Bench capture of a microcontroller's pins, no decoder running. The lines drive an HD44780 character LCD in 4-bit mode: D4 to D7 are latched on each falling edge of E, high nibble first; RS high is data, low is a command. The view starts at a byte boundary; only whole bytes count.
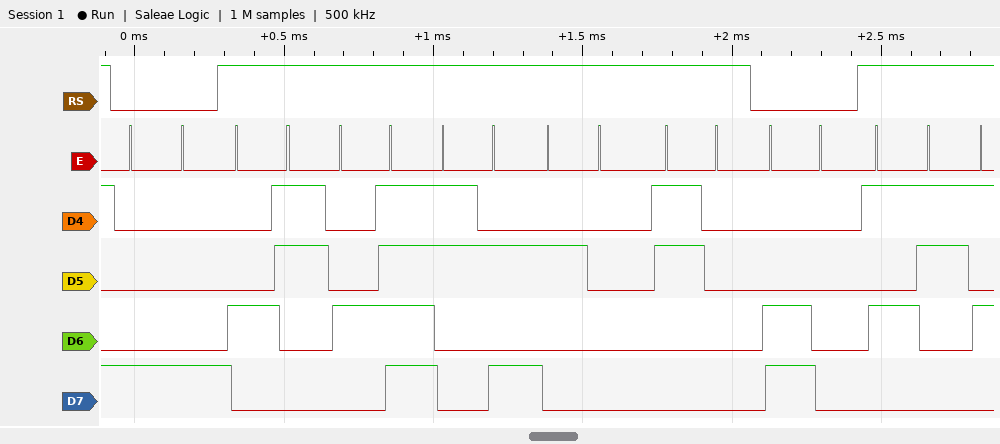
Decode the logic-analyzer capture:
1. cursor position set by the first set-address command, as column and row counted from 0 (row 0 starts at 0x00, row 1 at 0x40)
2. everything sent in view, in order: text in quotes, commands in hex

column 8, row 0
0x88 "CO: 0" 0xC0 "S"
